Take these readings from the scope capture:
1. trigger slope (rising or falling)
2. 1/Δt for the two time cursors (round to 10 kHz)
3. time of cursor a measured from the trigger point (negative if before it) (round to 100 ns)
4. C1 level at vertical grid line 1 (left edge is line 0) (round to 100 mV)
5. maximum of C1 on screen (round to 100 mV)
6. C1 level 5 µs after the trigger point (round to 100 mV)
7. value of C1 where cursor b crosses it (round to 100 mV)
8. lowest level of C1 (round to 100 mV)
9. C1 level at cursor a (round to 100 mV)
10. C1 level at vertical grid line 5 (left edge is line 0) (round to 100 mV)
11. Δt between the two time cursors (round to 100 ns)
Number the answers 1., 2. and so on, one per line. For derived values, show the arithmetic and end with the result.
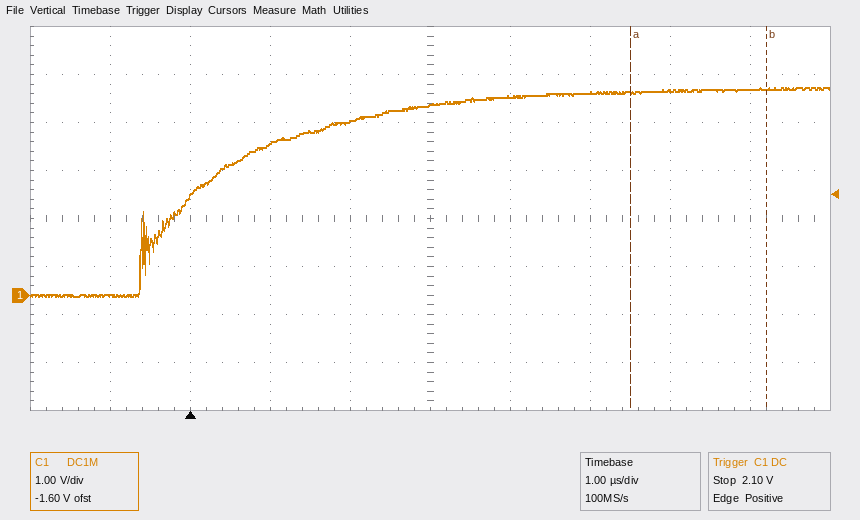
1. rising
2. 1 / 1.7 µs ≈ 590 kHz
3. +5.5 µs
4. 0.0 V
5. 4.3 V
6. 4.2 V
7. 4.3 V
8. 0.0 V
9. 4.2 V
10. 4.0 V
11. 1.7 µs
